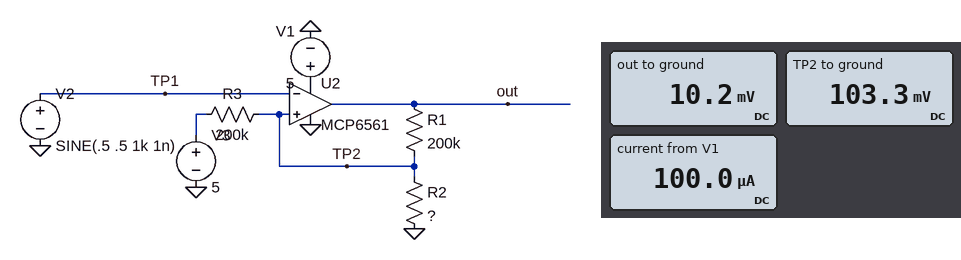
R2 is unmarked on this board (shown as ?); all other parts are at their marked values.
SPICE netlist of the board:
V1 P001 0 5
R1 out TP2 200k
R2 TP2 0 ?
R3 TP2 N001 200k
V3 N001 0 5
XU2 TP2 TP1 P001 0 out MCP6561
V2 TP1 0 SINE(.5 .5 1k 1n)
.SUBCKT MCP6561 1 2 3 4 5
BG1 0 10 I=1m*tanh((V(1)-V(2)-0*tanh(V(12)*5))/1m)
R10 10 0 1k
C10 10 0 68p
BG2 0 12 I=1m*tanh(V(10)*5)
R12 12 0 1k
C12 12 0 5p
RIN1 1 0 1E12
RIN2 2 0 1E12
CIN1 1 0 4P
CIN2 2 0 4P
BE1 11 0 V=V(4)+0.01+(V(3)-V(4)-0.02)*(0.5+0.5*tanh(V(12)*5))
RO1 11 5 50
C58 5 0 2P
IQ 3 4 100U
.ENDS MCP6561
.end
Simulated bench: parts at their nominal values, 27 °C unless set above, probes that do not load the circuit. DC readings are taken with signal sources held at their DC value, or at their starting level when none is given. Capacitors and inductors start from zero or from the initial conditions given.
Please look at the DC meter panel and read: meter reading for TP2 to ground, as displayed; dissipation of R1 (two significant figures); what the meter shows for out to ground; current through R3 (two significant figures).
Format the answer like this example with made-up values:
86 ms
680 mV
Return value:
103.3 mV
43 nW
10.2 mV
24 µA
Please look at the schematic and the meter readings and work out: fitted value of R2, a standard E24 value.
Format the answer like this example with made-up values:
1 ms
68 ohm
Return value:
4.3 kΩ
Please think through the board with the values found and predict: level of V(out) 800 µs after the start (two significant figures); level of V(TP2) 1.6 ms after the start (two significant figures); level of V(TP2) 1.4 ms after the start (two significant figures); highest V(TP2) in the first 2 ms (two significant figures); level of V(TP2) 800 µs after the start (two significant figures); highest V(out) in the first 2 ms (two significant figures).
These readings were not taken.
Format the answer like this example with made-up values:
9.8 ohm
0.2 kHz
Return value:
5.0 V
100 mV
100 mV
210 mV
210 mV
5.0 V
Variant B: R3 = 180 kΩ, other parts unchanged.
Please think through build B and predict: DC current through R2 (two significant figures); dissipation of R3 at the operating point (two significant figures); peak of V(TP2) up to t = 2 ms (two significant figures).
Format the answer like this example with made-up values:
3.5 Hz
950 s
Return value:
27 µA
130 µW
220 mV
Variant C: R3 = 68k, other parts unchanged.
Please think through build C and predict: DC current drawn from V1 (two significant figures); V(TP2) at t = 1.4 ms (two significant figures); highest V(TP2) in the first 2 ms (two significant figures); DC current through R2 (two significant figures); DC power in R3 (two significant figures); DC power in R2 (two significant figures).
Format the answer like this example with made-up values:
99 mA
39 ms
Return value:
100 µA
290 mV
390 mV
68 µA
330 µW
20 µW
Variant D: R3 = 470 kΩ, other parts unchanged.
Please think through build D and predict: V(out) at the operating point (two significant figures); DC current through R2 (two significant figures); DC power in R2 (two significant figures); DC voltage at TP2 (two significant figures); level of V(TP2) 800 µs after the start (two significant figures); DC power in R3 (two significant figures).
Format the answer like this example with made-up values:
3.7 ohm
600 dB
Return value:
10 mV
10 µA
460 nW
45 mV
150 mV
52 µW
